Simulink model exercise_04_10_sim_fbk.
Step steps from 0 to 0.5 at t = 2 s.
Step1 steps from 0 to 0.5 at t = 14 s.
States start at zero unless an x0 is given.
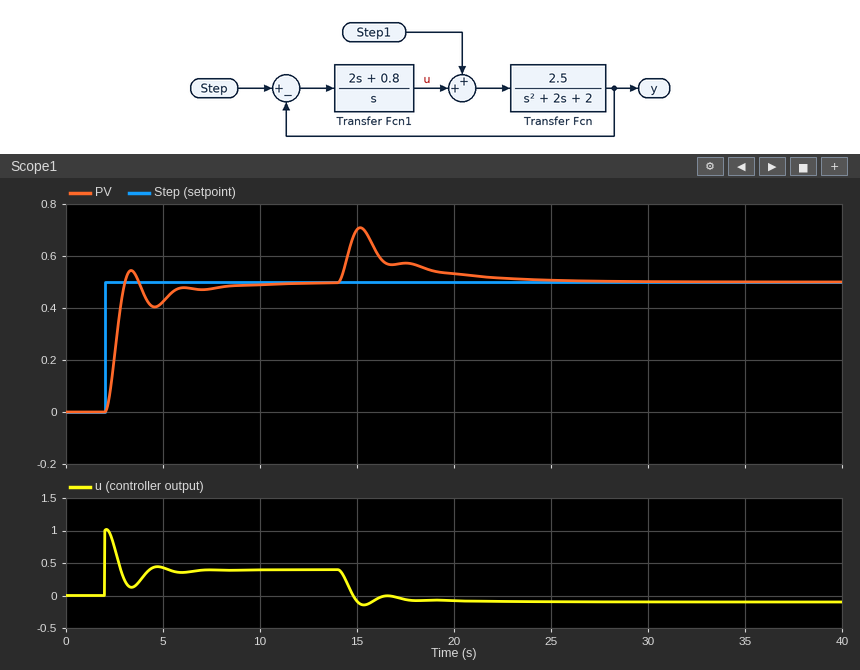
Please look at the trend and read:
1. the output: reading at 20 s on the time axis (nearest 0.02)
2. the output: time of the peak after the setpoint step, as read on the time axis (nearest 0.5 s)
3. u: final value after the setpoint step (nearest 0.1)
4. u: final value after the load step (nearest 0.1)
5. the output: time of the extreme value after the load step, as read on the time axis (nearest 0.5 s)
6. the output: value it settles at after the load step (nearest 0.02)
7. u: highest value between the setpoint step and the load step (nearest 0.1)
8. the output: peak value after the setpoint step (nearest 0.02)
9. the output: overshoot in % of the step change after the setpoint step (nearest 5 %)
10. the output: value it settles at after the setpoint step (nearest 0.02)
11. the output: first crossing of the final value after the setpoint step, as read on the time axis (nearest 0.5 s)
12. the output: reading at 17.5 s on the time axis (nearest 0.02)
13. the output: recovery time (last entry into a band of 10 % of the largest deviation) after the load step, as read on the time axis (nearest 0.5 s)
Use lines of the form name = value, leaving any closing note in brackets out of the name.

the output: reading at 20 s on the time axis = 0.54
the output: time of the peak after the setpoint step, as read on the time axis = 3.5 s
u: final value after the setpoint step = 0.4
u: final value after the load step = -0.1
the output: time of the extreme value after the load step, as read on the time axis = 15.0 s
the output: value it settles at after the load step = 0.50
u: highest value between the setpoint step and the load step = 1.0
the output: peak value after the setpoint step = 0.54
the output: overshoot in % of the step change after the setpoint step = 10 %
the output: value it settles at after the setpoint step = 0.50
the output: first crossing of the final value after the setpoint step, as read on the time axis = 3.0 s
the output: reading at 17.5 s on the time axis = 0.58
the output: recovery time (last entry into a band of 10 % of the largest deviation) after the load step, as read on the time axis = 21.5 s
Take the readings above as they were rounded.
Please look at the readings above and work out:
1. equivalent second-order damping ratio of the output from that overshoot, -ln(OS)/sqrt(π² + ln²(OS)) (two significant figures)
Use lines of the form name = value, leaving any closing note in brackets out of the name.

equivalent second-order damping ratio of the output from that overshoot, -ln(OS)/sqrt(π² + ln²(OS)) = 0.59
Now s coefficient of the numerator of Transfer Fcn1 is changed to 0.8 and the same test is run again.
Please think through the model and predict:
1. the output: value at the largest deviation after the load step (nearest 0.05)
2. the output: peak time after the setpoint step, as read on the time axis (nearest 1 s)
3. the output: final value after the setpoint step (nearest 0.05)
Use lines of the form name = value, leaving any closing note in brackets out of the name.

the output: value at the largest deviation after the load step = 0.80
the output: peak time after the setpoint step, as read on the time axis = 4 s
the output: final value after the setpoint step = 0.50
